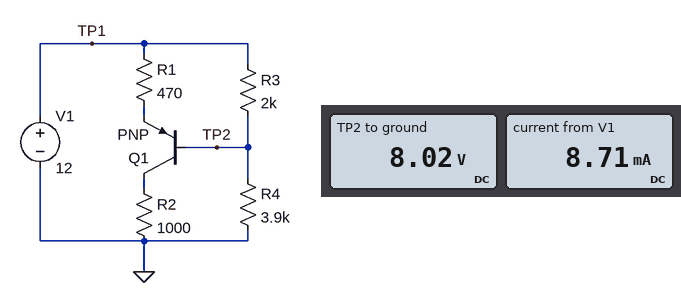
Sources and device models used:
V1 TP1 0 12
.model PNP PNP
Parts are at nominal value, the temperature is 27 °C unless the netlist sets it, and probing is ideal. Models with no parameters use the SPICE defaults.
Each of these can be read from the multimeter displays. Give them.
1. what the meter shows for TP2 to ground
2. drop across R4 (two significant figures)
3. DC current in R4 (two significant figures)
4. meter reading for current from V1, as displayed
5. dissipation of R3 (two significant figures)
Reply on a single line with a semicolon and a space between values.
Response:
8.02 V; 8.0 V; 2.1 mA; 8.71 mA; 7.9 mW
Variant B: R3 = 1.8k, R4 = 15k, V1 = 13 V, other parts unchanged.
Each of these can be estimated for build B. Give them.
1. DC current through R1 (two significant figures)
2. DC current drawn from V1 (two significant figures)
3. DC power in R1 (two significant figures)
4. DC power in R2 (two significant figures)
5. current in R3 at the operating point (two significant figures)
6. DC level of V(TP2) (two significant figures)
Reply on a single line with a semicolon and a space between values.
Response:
1.3 mA; 2.0 mA; 750 µW; 1.6 mW; 760 µA; 12 V
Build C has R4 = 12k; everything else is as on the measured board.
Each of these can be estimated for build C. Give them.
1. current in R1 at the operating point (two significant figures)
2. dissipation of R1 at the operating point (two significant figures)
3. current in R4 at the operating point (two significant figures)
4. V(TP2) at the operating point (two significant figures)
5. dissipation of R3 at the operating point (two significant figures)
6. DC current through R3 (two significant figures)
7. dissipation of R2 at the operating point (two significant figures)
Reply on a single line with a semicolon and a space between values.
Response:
1.9 mA; 1.7 mW; 860 µA; 10 V; 1.4 mW; 840 µA; 3.5 mW
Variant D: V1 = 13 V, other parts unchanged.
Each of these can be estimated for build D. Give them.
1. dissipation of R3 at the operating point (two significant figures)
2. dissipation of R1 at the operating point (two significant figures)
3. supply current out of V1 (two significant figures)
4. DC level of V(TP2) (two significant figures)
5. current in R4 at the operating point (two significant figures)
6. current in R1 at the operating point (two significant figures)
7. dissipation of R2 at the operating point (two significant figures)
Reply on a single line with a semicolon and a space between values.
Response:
9.3 mW; 26 mW; 9.6 mA; 8.7 V; 2.2 mA; 7.4 mA; 54 mW
